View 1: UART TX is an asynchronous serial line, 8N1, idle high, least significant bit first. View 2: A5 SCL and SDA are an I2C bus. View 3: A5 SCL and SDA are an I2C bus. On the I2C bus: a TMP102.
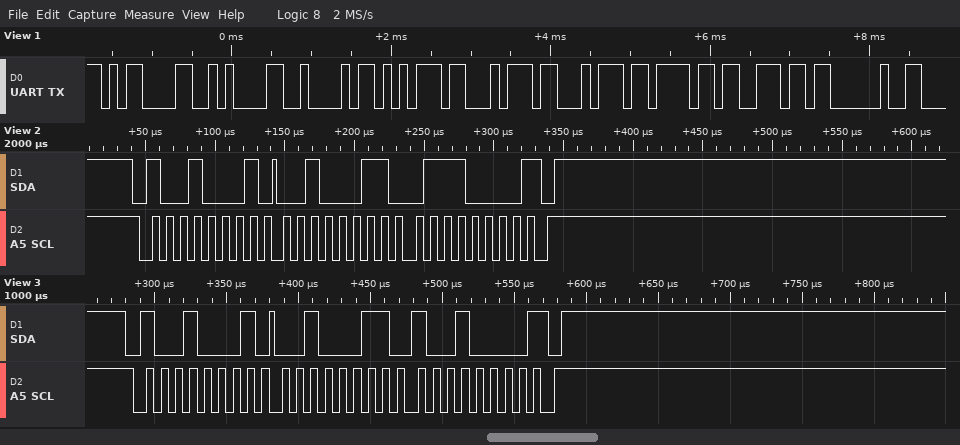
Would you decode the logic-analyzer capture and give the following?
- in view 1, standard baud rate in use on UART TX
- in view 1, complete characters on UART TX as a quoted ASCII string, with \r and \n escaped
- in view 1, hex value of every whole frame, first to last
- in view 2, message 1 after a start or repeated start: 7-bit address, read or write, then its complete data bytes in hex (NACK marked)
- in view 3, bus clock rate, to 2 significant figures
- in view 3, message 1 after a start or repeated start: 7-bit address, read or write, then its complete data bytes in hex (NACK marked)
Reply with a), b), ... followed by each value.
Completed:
a) 9600 baud
b) "\r\nButton "
c) 0x0D 0x0A 0x42 0x75 0x74 0x74 0x6F 0x6E 0x20
d) 0x48 read: 23 70 NACK
e) 100 kHz
f) 0x48 read: 23 90 NACK
